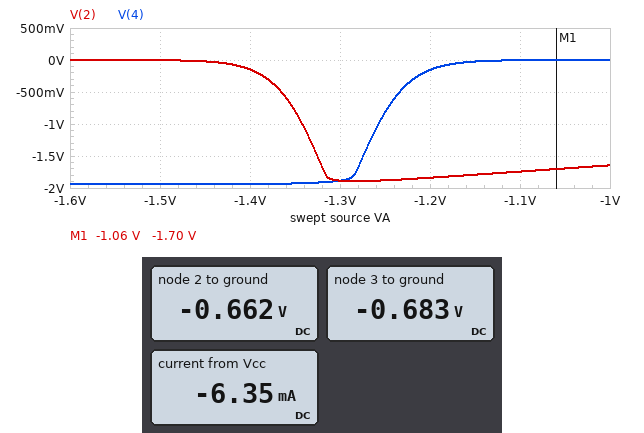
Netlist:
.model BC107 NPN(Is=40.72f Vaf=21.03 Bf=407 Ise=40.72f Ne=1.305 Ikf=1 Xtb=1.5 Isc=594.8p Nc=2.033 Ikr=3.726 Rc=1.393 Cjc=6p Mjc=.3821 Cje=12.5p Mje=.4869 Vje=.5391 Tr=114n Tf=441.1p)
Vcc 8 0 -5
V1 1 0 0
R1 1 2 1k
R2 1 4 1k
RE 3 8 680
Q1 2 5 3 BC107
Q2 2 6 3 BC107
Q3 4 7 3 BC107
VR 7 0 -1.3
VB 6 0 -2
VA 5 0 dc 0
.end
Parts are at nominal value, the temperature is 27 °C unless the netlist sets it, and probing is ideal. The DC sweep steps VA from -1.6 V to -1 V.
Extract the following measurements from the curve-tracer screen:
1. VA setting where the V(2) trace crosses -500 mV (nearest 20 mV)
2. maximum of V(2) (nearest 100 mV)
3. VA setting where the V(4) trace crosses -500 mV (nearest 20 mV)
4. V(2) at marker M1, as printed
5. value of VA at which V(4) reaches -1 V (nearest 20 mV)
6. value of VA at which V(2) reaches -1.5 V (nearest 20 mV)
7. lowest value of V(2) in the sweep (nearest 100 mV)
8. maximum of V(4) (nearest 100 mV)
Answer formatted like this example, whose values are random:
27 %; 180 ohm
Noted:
-1.36 V; 0 V; -1.24 V; -1.70 V; -1.26 V; -1.32 V; -1.9 V; 0 V
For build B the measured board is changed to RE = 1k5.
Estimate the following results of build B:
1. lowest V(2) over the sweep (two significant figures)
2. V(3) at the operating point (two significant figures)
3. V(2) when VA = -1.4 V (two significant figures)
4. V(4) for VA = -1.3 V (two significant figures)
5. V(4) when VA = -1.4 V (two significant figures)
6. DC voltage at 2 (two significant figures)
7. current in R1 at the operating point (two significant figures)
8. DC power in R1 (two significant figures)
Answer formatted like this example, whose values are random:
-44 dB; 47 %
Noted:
-1.8 V; -660 mV; -48 mV; -1.0 V; -1.9 V; -640 mV; 640 µA; 410 µW
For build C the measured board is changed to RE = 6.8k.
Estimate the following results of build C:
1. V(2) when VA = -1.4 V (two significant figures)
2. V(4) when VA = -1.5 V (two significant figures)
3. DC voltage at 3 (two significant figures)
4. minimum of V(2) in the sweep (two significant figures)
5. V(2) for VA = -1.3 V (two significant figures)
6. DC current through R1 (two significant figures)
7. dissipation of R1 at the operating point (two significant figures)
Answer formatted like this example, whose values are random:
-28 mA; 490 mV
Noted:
-9.5 mV; -450 mV; -610 mV; -500 mV; -230 mV; 550 µA; 300 µW
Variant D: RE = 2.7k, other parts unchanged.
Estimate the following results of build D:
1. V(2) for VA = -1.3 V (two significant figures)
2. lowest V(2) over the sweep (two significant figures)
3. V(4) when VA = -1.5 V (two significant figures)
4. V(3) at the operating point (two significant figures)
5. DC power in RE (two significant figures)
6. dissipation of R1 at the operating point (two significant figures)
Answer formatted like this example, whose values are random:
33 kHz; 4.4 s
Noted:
-570 mV; -1.2 V; -1.1 V; -640 mV; 7.0 mW; 380 µW
